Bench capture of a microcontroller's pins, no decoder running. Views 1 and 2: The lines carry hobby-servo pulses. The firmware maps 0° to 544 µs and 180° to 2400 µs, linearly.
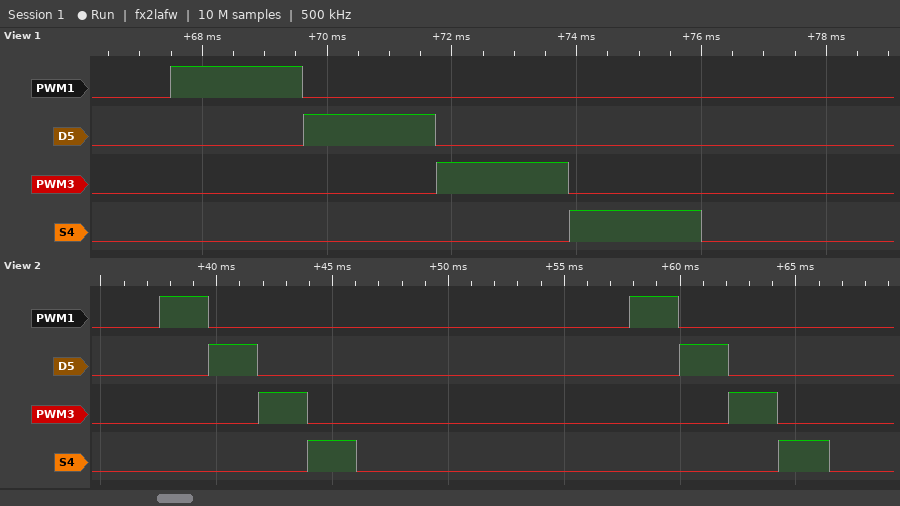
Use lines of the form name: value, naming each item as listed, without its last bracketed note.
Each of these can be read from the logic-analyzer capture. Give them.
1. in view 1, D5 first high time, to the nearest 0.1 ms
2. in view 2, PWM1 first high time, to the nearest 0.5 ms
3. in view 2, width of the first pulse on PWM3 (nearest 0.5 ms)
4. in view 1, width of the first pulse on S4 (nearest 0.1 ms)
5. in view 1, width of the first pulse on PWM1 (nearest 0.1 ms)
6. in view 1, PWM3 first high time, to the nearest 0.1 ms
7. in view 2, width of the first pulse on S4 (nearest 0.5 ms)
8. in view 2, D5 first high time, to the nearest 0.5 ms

in view 1, D5 first high time, to the nearest 0.1 ms: 2.1 ms
in view 2, PWM1 first high time, to the nearest 0.5 ms: 2.0 ms
in view 2, width of the first pulse on PWM3: 2.0 ms
in view 1, width of the first pulse on S4: 2.1 ms
in view 1, width of the first pulse on PWM1: 2.1 ms
in view 1, PWM3 first high time, to the nearest 0.1 ms: 2.1 ms
in view 2, width of the first pulse on S4: 2.0 ms
in view 2, D5 first high time, to the nearest 0.5 ms: 2.0 ms
